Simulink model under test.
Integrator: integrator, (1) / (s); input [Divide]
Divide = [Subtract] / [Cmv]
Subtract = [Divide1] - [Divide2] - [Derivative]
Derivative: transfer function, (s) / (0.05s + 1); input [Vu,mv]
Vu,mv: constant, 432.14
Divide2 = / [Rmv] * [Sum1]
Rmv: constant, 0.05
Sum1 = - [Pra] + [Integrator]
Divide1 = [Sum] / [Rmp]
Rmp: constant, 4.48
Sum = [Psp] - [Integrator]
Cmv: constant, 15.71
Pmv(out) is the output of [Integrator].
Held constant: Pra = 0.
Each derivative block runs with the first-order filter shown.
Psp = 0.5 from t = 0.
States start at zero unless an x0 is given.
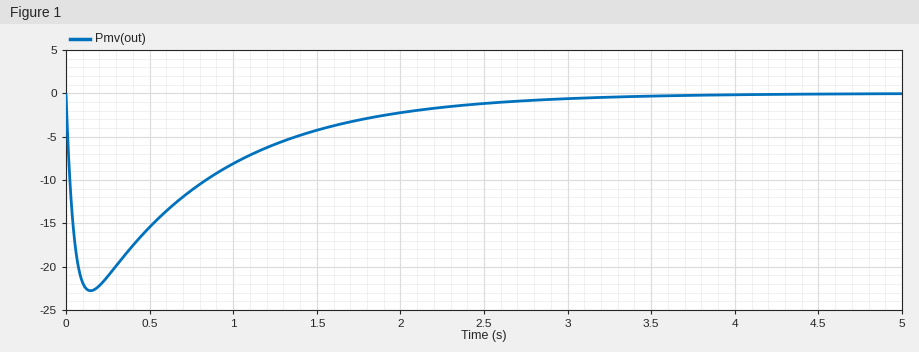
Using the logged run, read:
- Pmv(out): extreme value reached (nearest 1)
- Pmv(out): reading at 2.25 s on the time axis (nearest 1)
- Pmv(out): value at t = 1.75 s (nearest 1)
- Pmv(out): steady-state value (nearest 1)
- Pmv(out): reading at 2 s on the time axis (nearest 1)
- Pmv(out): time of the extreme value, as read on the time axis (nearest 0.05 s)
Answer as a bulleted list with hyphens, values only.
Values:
- -23
- -2
- -3
- 0
- -2
- 0.15 s
